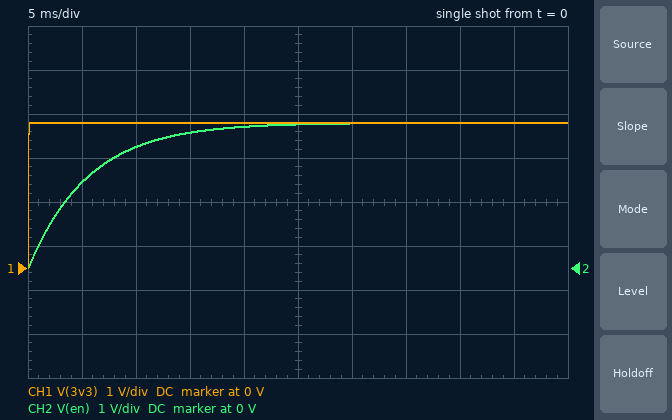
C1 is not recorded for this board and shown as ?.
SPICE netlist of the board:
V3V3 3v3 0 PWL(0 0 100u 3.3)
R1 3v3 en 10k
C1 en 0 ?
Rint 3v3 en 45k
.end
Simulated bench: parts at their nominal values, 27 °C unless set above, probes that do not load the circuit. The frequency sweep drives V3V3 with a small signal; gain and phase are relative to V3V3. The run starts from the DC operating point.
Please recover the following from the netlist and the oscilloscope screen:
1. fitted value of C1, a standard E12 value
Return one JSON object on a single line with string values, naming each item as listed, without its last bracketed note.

{"fitted value of C1, a standard E12 value": "680 nF"}
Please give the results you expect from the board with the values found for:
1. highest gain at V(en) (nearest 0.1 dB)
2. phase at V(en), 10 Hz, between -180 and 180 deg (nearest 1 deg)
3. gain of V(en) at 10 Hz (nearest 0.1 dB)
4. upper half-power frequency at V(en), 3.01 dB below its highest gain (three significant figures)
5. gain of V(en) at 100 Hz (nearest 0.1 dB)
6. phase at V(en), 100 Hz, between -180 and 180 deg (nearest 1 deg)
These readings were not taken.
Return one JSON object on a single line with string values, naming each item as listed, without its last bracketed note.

{"highest gain at V(en)": "0 dB", "phase at V(en), 10 Hz, between -180 and 180 deg": "-19 deg", "gain of V(en) at 10 Hz": "-0.5 dB", "upper half-power frequency at V(en), 3.01 dB below its highest gain": "28.6 Hz", "gain of V(en) at 100 Hz": "-11.2 dB", "phase at V(en), 100 Hz, between -180 and 180 deg": "-74 deg"}
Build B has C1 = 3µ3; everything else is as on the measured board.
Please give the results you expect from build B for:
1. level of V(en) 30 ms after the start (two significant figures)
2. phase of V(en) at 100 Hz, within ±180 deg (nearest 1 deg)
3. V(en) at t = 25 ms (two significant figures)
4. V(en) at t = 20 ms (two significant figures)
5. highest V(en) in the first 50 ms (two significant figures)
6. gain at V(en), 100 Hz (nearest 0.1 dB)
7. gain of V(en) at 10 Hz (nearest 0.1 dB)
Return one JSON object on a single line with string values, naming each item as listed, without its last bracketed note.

{"level of V(en) 30 ms after the start": "2.2 V", "phase of V(en) at 100 Hz, within ±180 deg": "-87 deg", "V(en) at t = 25 ms": "2.0 V", "V(en) at t = 20 ms": "1.7 V", "highest V(en) in the first 50 ms": "2.8 V", "gain at V(en), 100 Hz": "-24.6 dB", "gain of V(en) at 10 Hz": "-5.9 dB"}
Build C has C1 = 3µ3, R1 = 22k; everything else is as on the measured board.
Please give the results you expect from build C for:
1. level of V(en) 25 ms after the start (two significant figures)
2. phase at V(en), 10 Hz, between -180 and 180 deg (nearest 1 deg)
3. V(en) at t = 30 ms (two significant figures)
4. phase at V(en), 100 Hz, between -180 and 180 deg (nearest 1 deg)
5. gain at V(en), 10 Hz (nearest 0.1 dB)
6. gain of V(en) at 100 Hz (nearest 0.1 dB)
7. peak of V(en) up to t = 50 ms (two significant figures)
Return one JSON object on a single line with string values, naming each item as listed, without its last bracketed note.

{"level of V(en) 25 ms after the start": "1.3 V", "phase at V(en), 10 Hz, between -180 and 180 deg": "-72 deg", "V(en) at t = 30 ms": "1.5 V", "phase at V(en), 100 Hz, between -180 and 180 deg": "-88 deg", "gain at V(en), 10 Hz": "-10.2 dB", "gain of V(en) at 100 Hz": "-29.7 dB", "peak of V(en) up to t = 50 ms": "2.1 V"}
